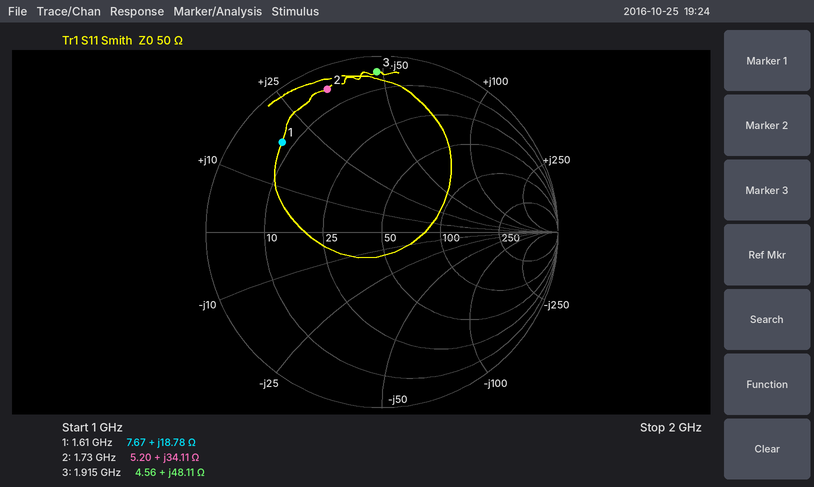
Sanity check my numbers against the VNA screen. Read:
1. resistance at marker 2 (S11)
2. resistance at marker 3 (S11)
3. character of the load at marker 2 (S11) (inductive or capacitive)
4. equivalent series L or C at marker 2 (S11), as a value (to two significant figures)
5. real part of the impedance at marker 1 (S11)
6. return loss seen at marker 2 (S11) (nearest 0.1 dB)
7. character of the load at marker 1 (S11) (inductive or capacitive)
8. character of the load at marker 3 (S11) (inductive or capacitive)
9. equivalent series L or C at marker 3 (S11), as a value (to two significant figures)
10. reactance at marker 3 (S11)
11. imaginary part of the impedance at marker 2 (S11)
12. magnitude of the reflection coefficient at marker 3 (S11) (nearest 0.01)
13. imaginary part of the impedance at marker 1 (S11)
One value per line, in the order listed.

5.20 Ω
4.56 Ω
inductive
3.1 nH
7.67 Ω
1.2 dB
inductive
inductive
4.0 nH
+48.11 Ω
+34.11 Ω
0.91
+18.78 Ω
